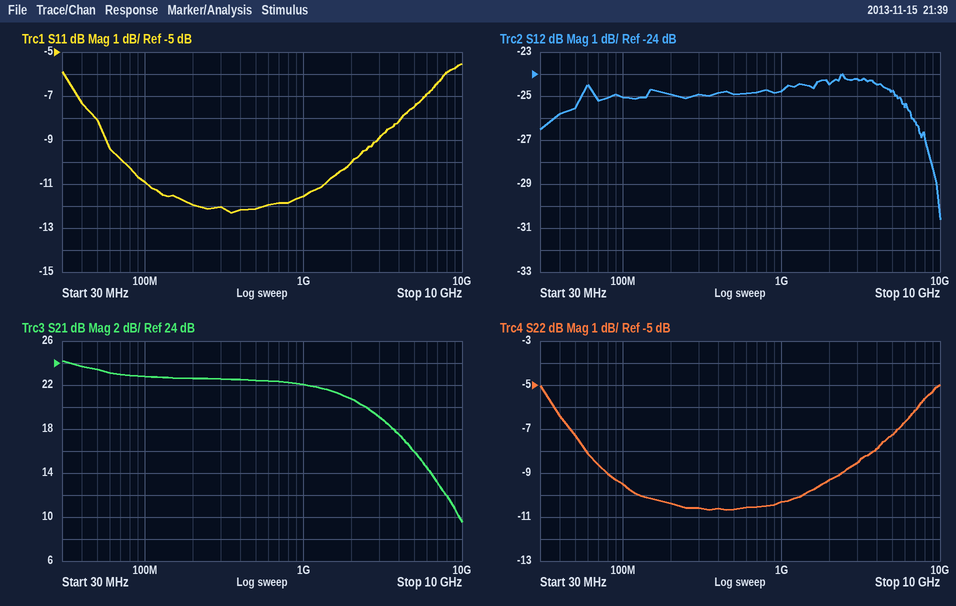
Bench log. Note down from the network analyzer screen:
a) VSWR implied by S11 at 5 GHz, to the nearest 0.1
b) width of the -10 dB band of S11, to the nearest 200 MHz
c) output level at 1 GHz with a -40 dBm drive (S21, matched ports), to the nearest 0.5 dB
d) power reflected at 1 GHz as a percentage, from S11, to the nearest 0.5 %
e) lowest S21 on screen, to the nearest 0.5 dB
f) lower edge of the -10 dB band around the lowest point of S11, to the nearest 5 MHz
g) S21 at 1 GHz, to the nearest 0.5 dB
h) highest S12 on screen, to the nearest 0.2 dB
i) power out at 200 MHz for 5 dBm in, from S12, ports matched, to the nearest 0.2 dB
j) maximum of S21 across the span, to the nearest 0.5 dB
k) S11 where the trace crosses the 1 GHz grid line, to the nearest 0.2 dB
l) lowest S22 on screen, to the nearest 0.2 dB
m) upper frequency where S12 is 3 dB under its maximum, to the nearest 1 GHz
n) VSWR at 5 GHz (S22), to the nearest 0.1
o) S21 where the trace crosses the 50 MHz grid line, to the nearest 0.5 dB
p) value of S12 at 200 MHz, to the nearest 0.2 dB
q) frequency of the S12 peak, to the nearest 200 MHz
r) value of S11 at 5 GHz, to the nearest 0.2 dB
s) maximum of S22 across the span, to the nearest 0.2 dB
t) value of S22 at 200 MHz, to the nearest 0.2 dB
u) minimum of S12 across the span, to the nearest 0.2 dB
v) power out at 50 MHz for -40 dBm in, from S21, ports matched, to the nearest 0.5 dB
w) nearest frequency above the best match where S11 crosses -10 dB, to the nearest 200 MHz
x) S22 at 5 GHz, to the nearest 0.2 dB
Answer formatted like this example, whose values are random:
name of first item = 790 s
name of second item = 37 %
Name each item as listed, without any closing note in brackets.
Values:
VSWR implied by S11 at 5 GHz, to the nearest 0.1 = 2.5
width of the -10 dB band of S11, to the nearest 200 MHz = 2.0 GHz
output level at 1 GHz with a -40 dBm drive (S21, matched ports), to the nearest 0.5 dB = -18.0 dBm
power reflected at 1 GHz as a percentage, from S11, to the nearest 0.5 % = 7.0 %
lowest S21 on screen, to the nearest 0.5 dB = 9.5 dB
lower edge of the -10 dB band around the lowest point of S11, to the nearest 5 MHz = 75 MHz
S21 at 1 GHz, to the nearest 0.5 dB = 22.0 dB
highest S12 on screen, to the nearest 0.2 dB = -24.0 dB
power out at 200 MHz for 5 dBm in, from S12, ports matched, to the nearest 0.2 dB = -20.0 dBm
maximum of S21 across the span, to the nearest 0.5 dB = 24.0 dB
S11 where the trace crosses the 1 GHz grid line, to the nearest 0.2 dB = -11.6 dB
lowest S22 on screen, to the nearest 0.2 dB = -10.6 dB
upper frequency where S12 is 3 dB under its maximum, to the nearest 1 GHz = 8 GHz
VSWR at 5 GHz (S22), to the nearest 0.1 = 2.5
S21 where the trace crosses the 50 MHz grid line, to the nearest 0.5 dB = 23.5 dB
value of S12 at 200 MHz, to the nearest 0.2 dB = -25.0 dB
frequency of the S12 peak, to the nearest 200 MHz = 2.4 GHz
value of S11 at 5 GHz, to the nearest 0.2 dB = -7.4 dB
maximum of S22 across the span, to the nearest 0.2 dB = -5.0 dB
value of S22 at 200 MHz, to the nearest 0.2 dB = -10.4 dB
minimum of S12 across the span, to the nearest 0.2 dB = -30.6 dB
power out at 50 MHz for -40 dBm in, from S21, ports matched, to the nearest 0.5 dB = -16.5 dBm
nearest frequency above the best match where S11 crosses -10 dB, to the nearest 200 MHz = 2.0 GHz
S22 at 5 GHz, to the nearest 0.2 dB = -7.2 dB
